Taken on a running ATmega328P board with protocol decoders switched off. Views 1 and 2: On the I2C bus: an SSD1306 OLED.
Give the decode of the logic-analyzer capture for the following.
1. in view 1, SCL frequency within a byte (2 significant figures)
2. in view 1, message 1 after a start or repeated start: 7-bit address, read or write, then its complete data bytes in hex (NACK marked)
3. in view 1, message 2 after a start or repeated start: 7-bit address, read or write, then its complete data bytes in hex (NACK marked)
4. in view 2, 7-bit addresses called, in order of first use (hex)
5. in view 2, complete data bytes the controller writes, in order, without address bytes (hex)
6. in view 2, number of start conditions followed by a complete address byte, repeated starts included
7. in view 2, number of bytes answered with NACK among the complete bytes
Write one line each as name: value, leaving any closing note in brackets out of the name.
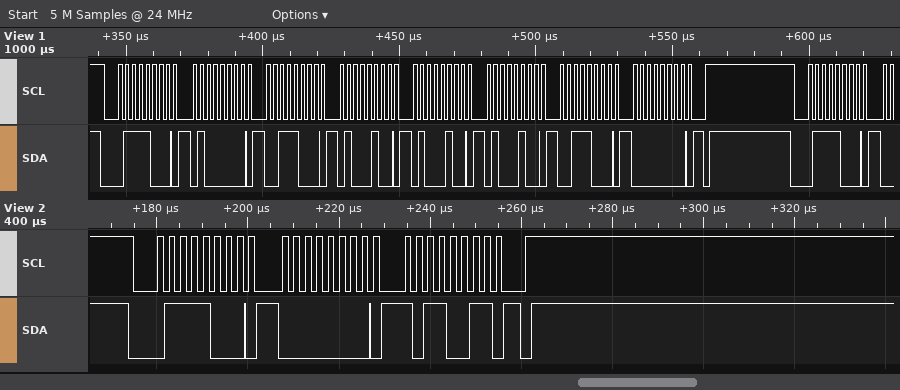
in view 1, SCL frequency within a byte: 400 kHz
in view 1, message 1 after a start or repeated start: 7-bit address, read or write, then its complete data bytes in hex: 0x3C write: 40 38 44 44 44 38 00
in view 1, message 2 after a start or repeated start: 7-bit address, read or write, then its complete data bytes in hex: 0x3C write
in view 2, 7-bit addresses called, in order of first use: 0x3C
in view 2, complete data bytes the controller writes, in order, without address bytes: 00 B3
in view 2, number of start conditions followed by a complete address byte, repeated starts included: 1
in view 2, number of bytes answered with NACK among the complete bytes: 0
